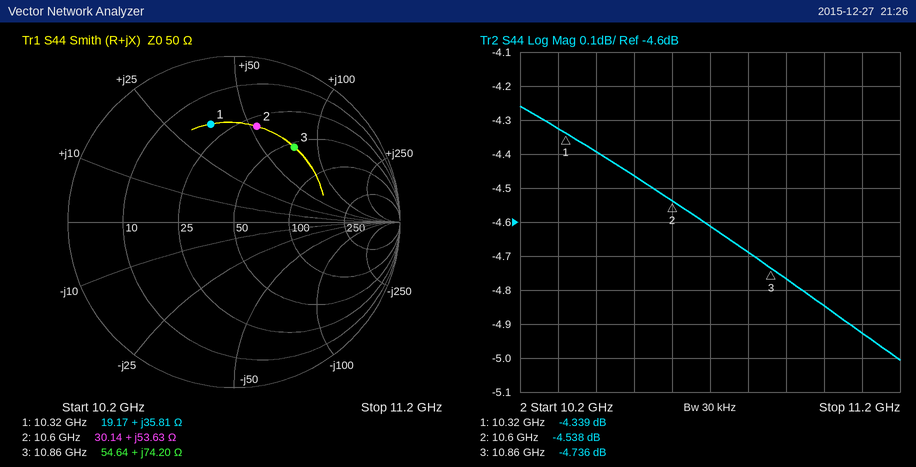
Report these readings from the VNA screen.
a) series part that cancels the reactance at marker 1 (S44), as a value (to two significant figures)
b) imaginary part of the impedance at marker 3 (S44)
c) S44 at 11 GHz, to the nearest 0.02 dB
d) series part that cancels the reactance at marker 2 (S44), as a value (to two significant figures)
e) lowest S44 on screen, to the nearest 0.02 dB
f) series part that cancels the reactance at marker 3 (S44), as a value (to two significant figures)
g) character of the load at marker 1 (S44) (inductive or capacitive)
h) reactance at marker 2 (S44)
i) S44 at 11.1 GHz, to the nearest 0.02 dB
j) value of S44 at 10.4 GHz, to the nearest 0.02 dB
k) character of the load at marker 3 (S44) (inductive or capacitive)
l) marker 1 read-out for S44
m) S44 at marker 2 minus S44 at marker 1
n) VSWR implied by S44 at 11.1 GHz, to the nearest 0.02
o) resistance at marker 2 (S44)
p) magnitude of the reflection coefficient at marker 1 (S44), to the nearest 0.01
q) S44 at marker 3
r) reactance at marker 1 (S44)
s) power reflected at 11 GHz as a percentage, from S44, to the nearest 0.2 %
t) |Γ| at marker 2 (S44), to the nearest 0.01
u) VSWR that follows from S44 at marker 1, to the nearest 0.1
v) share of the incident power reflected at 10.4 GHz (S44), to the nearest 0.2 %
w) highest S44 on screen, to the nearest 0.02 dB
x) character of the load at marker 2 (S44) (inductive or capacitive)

430 fF
+74.20 Ω
-4.84 dB
280 fF
-5.00 dB
200 fF
inductive
+53.63 Ω
-4.92 dB
-4.40 dB
inductive
-4.339 dB
-0.199 dB
3.62
30.14 Ω
0.61
-4.736 dB
+35.81 Ω
32.8 %
0.59
4.1
36.4 %
-4.26 dB
inductive
